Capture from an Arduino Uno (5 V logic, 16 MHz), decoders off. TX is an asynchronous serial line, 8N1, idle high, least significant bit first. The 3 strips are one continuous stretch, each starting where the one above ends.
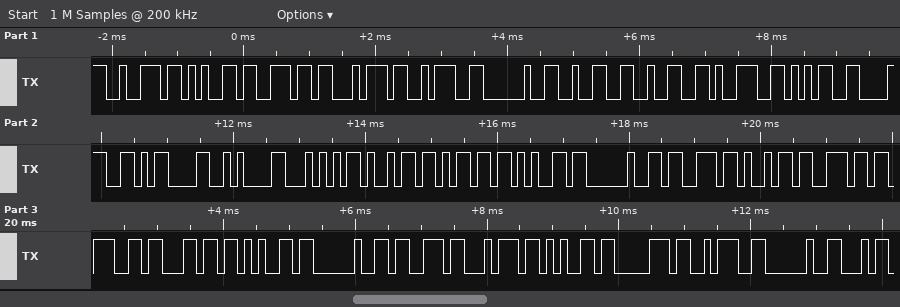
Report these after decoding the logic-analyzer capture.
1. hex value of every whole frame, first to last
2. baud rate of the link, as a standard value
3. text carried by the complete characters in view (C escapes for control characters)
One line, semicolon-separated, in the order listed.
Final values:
72 65 6E 74 3A 20 32 32 39 35 38 0D 0A 54 69 6D 65 20 73 69 6E 67 6C 65 20 73 74 65 70 3A 20; 9600 baud; "rent: 22958\r\nTime single step: "
